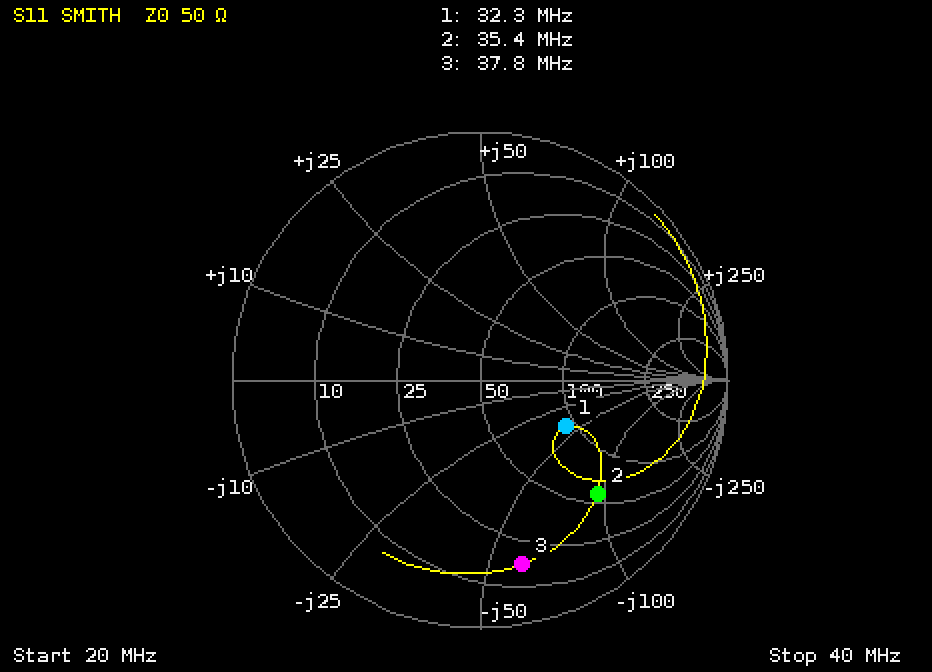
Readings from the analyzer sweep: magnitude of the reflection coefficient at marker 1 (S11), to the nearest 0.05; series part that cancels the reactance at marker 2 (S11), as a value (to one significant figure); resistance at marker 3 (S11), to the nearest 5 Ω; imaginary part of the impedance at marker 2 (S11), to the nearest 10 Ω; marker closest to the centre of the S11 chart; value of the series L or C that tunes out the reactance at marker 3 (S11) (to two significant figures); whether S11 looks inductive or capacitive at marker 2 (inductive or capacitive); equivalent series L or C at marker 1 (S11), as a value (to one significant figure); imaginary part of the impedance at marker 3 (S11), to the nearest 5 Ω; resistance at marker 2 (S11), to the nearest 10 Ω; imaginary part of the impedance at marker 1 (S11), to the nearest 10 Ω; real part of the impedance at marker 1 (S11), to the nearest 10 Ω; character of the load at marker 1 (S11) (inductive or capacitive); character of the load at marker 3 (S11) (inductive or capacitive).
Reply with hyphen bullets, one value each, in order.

- 0.40
- 400 nH
- 15 Ω
- -90 Ω
- marker 1
- 250 nH
- capacitive
- 100 pF
- -60 Ω
- 60 Ω
- -40 Ω
- 90 Ω
- capacitive
- capacitive
